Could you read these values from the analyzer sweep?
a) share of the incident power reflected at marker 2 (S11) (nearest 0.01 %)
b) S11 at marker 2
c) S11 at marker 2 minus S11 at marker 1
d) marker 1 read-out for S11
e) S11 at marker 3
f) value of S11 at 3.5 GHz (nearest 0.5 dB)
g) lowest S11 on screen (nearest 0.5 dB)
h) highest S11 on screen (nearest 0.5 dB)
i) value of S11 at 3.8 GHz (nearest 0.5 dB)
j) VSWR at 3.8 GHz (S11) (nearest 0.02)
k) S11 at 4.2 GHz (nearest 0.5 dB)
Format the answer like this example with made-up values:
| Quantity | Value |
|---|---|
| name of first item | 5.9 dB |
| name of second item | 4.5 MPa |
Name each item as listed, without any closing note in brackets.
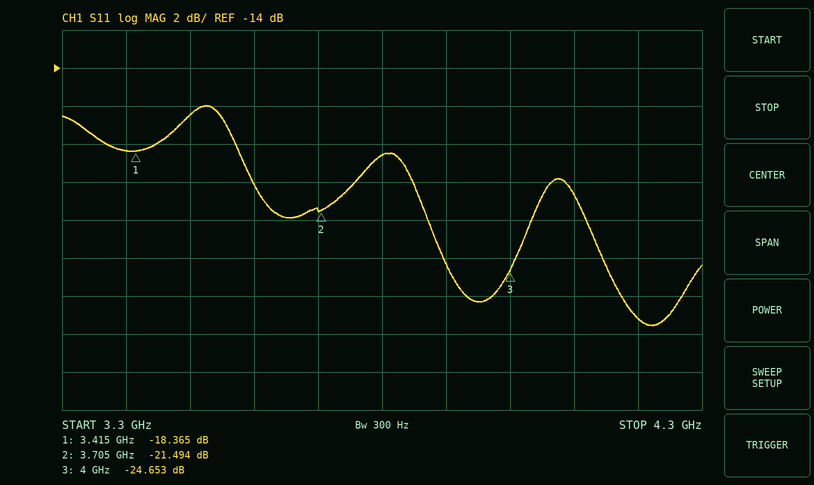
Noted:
| Quantity | Value |
|---|---|
| share of the incident power reflected at marker 2 (S11) | 0.71 % |
| S11 at marker 2 | -21.494 dB |
| S11 at marker 2 minus S11 at marker 1 | -3.129 dB |
| marker 1 read-out for S11 | -18.365 dB |
| S11 at marker 3 | -24.653 dB |
| value of S11 at 3.5 GHz | -16.5 dB |
| lowest S11 on screen | -27.5 dB |
| highest S11 on screen | -16.0 dB |
| value of S11 at 3.8 GHz | -18.5 dB |
| VSWR at 3.8 GHz (S11) | 1.26 |
| S11 at 4.2 GHz | -27.0 dB |
